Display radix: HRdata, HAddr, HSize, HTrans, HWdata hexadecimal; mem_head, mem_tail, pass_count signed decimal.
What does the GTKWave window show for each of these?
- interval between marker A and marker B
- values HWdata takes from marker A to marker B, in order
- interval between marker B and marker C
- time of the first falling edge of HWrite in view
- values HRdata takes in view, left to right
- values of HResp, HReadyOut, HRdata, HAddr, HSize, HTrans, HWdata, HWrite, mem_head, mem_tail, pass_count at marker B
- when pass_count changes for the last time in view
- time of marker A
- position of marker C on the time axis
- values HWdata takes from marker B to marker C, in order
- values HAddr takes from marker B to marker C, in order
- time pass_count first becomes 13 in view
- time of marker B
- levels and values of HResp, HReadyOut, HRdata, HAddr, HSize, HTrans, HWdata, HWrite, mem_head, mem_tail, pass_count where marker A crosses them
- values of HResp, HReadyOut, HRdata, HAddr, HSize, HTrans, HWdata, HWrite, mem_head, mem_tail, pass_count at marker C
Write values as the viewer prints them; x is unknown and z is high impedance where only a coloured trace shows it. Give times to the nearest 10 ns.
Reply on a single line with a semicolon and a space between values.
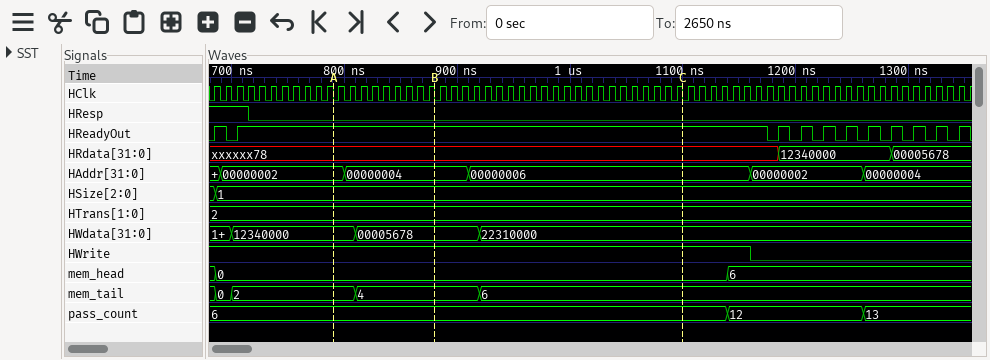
90 ns; 12340000, 00005678; 220 ns; 1160 ns; xxxxxx78, 12340000, 00005678; HResp=0, HReadyOut=1, HRdata=xxxxxx78, HAddr=00000004, HSize=1, HTrans=2, HWdata=00005678, HWrite=1, mem_head=0, mem_tail=4, pass_count=6; 1260 ns; 790 ns; 1100 ns; 00005678, 22310000; 00000004, 00000006; 1260 ns; 880 ns; HResp=0, HReadyOut=1, HRdata=xxxxxx78, HAddr=00000002, HSize=1, HTrans=2, HWdata=12340000, HWrite=1, mem_head=0, mem_tail=2, pass_count=6; HResp=0, HReadyOut=1, HRdata=xxxxxx78, HAddr=00000006, HSize=1, HTrans=2, HWdata=22310000, HWrite=1, mem_head=0, mem_tail=6, pass_count=6
